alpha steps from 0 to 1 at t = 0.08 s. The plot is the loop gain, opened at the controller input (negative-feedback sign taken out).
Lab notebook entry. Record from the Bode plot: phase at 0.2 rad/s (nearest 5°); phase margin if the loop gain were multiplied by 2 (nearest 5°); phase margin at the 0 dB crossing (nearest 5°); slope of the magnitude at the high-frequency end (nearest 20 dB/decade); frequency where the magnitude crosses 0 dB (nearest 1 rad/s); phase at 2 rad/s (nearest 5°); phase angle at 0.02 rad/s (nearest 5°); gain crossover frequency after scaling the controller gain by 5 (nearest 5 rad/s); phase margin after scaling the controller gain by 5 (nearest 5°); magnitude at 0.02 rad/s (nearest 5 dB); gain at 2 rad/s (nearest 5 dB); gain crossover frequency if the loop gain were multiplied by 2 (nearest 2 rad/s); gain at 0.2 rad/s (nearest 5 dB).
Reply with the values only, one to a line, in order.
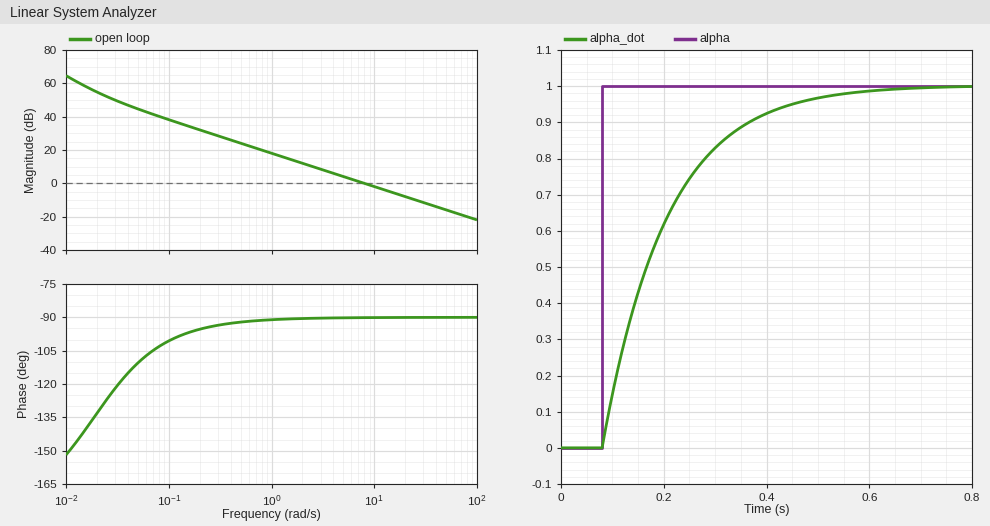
-95°
90°
90°
-20 dB/decade
8 rad/s
-90°
-135°
40 rad/s
90°
55 dB
10 dB
16 rad/s
30 dB
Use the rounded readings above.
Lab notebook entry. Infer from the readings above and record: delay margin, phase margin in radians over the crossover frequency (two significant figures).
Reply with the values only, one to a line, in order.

0.20 s
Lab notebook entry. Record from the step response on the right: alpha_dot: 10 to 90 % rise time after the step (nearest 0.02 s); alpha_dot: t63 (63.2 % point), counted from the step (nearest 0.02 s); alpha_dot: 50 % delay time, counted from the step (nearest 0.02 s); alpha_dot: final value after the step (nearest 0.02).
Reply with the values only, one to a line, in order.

0.28 s
0.12 s
0.08 s
1.00
